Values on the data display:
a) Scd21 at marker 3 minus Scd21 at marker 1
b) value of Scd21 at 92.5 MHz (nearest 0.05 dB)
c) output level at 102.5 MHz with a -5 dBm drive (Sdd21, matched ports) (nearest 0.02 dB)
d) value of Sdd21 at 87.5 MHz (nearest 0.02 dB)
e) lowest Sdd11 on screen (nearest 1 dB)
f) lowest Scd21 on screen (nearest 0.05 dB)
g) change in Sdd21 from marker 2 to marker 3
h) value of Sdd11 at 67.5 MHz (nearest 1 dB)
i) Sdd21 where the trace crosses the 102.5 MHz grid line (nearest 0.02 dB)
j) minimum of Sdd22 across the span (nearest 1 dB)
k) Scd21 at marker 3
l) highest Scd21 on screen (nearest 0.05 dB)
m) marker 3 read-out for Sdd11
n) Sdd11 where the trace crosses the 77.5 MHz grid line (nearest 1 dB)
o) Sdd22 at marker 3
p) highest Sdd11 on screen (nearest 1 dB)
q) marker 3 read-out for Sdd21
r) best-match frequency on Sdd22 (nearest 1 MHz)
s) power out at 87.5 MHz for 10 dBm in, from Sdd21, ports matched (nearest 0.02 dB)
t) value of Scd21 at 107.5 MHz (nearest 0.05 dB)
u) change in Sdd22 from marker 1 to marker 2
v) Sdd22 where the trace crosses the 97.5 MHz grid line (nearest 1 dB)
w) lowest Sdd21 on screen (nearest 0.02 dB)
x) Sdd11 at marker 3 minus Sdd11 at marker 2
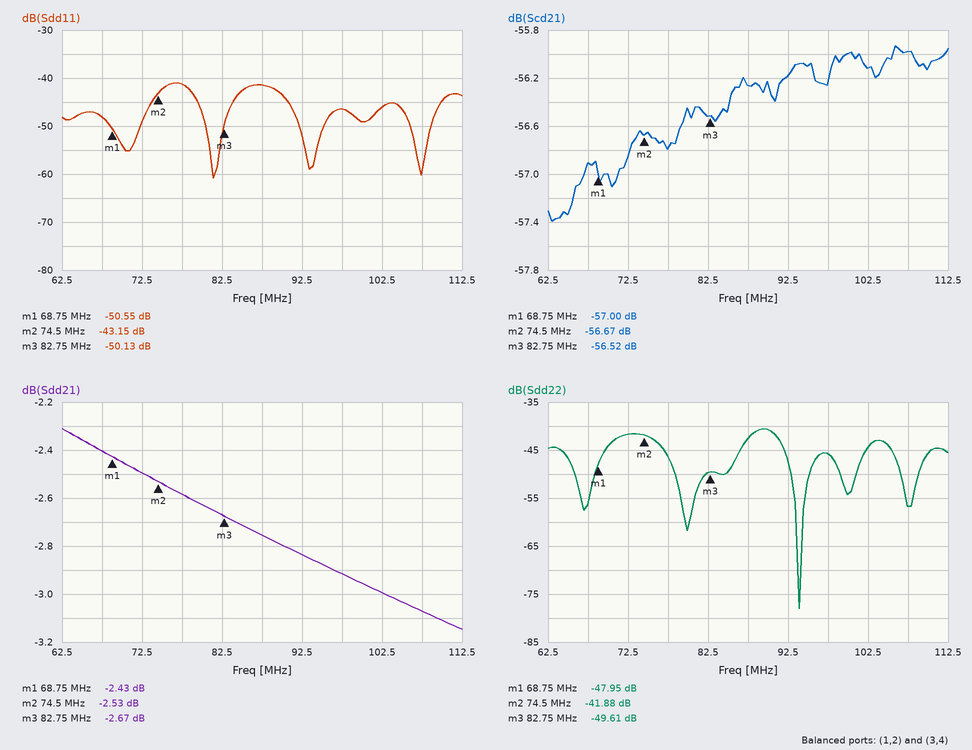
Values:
0.48 dB
-56.20 dB
-8.00 dBm
-2.76 dB
-61 dB
-57.40 dB
-0.14 dB
-48 dB
-3.00 dB
-78 dB
-56.52 dB
-55.95 dB
-50.13 dB
-41 dB
-49.61 dB
-41 dB
-2.67 dB
94 MHz
7.24 dBm
-56.00 dB
6.07 dB
-46 dB
-3.14 dB
-6.98 dB
